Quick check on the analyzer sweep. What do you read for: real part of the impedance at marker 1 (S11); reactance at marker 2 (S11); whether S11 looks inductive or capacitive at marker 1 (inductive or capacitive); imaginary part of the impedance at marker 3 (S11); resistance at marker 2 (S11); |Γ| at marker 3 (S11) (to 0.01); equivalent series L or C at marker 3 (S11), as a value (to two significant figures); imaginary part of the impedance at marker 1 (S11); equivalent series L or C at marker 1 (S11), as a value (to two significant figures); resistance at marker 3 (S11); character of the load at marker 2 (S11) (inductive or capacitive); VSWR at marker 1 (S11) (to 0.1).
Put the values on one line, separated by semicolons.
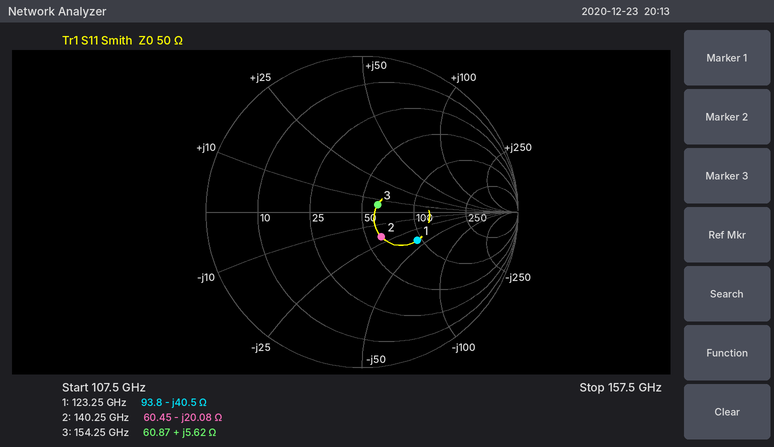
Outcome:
93.8 Ω; -20.08 Ω; capacitive; +5.62 Ω; 60.45 Ω; 0.11; 5.8 pH; -40.5 Ω; 32 fF; 60.87 Ω; capacitive; 2.3
